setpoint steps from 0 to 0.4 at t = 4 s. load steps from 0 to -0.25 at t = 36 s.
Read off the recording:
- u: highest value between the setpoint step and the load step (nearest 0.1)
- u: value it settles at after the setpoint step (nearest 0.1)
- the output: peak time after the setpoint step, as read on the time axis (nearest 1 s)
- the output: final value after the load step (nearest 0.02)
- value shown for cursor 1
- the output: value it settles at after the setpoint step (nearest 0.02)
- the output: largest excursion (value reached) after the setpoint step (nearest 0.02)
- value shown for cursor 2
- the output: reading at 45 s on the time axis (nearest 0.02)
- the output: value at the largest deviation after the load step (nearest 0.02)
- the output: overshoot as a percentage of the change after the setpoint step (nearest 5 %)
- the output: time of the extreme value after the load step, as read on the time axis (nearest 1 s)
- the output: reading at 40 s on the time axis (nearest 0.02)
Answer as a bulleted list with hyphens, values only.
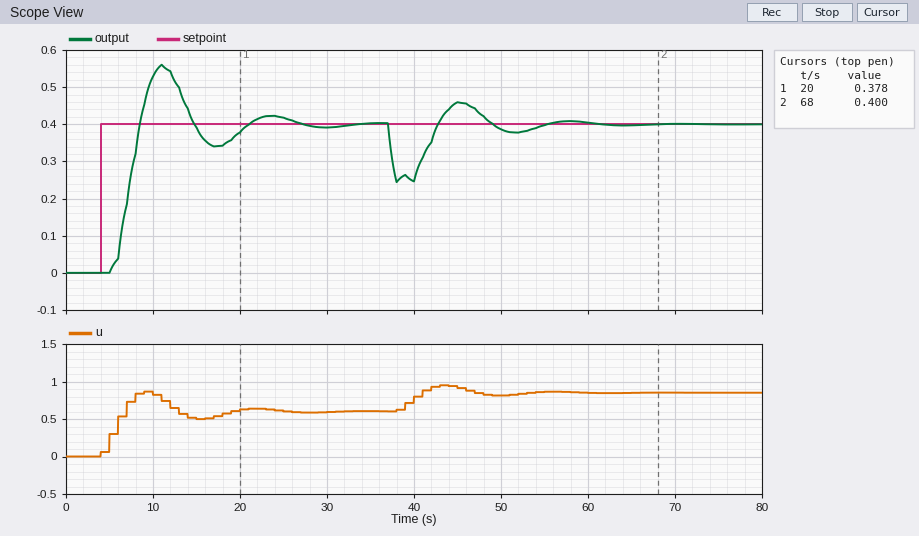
- 0.9
- 0.6
- 11 s
- 0.40
- 0.378
- 0.40
- 0.56
- 0.400
- 0.46
- 0.24
- 40 %
- 38 s
- 0.24
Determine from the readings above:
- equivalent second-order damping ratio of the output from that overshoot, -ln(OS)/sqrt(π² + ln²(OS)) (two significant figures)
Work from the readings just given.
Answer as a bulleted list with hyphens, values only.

- 0.28
